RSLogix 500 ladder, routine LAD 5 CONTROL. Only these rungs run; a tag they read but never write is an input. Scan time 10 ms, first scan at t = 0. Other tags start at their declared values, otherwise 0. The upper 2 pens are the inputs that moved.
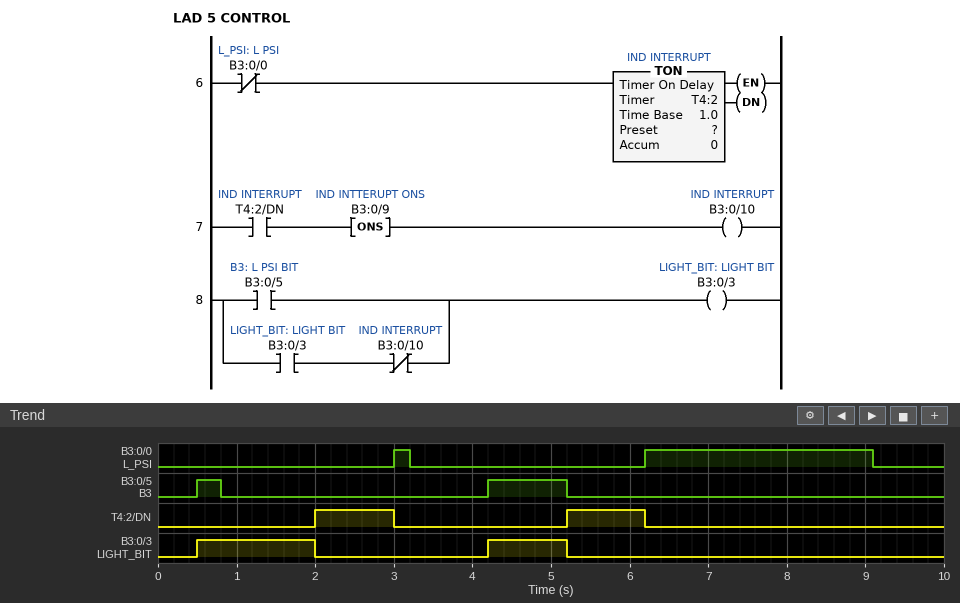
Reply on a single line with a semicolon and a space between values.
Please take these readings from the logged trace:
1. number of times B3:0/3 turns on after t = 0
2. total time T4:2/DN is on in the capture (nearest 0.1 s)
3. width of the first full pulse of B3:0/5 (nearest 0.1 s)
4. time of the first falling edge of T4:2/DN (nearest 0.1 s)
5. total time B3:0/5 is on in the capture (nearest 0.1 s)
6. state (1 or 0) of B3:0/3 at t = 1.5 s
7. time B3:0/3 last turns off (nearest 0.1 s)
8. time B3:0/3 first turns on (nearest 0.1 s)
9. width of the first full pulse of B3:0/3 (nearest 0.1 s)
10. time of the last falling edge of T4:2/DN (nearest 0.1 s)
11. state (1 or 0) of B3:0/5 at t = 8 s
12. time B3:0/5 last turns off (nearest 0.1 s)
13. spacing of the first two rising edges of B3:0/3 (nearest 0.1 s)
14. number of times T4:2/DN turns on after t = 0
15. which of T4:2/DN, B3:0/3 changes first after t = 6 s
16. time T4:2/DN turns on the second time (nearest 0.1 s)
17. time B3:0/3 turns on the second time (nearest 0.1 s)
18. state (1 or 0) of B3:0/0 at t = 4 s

2; 2.0 s; 0.3 s; 3.0 s; 1.3 s; 1; 5.2 s; 0.5 s; 1.5 s; 6.2 s; 0; 5.2 s; 3.7 s; 2; T4:2/DN; 5.2 s; 4.2 s; 0
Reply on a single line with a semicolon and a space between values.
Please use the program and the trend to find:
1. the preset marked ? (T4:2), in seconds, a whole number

2 s
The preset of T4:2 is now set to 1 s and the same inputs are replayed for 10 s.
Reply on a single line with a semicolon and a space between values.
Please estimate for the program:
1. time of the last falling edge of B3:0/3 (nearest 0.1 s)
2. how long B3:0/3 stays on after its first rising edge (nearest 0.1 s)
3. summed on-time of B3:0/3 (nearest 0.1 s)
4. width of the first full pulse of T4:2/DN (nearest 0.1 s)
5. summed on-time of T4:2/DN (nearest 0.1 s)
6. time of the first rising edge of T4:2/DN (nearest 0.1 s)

1.0 s; 0.5 s; 6.3 s; 2.0 s; 4.0 s; 1.0 s
